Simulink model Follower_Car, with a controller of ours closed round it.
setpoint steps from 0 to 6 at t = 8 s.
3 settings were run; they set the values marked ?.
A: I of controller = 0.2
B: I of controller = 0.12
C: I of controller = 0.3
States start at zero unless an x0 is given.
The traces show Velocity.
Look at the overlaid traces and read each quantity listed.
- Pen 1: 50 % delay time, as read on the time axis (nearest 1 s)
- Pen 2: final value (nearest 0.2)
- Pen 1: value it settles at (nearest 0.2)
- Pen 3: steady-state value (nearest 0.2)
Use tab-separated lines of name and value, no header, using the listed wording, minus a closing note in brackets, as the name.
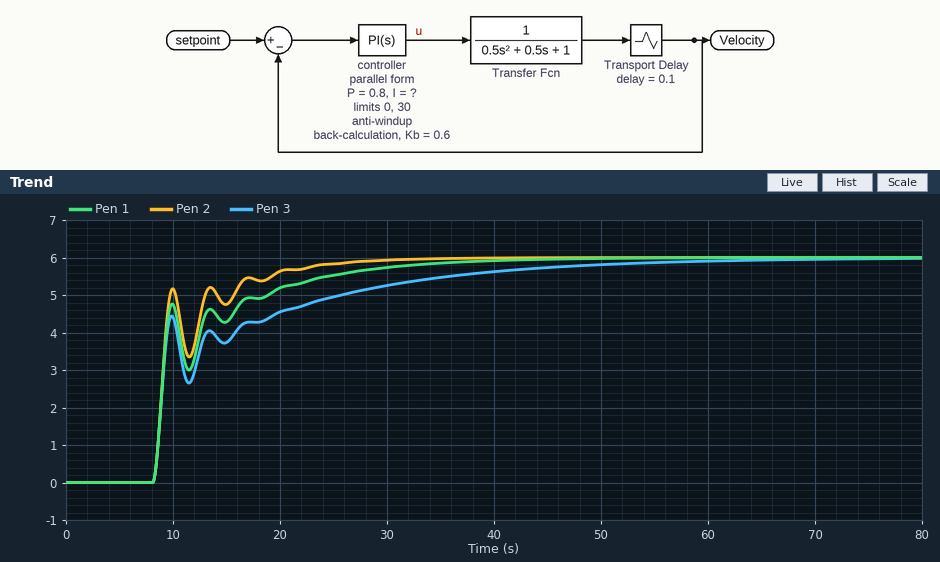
Pen 1: 50 % delay time, as read on the time axis	9 s
Pen 2: final value	6.0
Pen 1: value it settles at	6.0
Pen 3: steady-state value	6.0
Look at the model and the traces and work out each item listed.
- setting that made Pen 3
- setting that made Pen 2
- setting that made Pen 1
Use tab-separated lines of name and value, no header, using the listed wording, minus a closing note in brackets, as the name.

setting that made Pen 3	B
setting that made Pen 2	C
setting that made Pen 1	A
